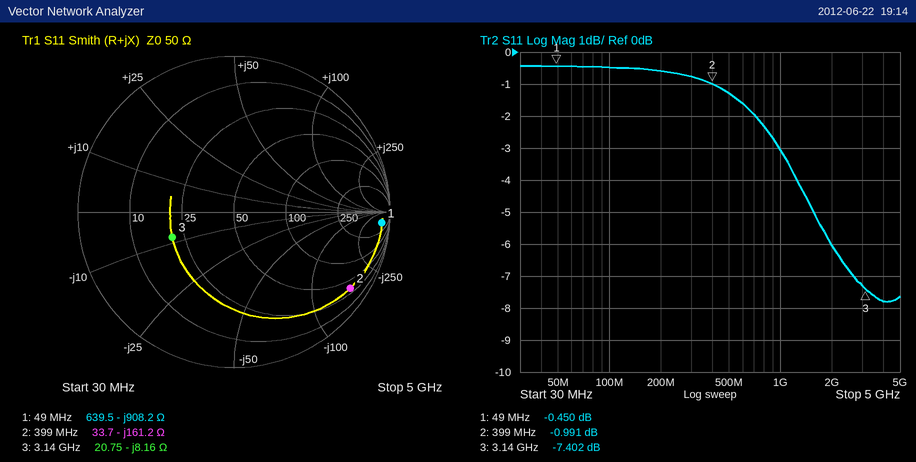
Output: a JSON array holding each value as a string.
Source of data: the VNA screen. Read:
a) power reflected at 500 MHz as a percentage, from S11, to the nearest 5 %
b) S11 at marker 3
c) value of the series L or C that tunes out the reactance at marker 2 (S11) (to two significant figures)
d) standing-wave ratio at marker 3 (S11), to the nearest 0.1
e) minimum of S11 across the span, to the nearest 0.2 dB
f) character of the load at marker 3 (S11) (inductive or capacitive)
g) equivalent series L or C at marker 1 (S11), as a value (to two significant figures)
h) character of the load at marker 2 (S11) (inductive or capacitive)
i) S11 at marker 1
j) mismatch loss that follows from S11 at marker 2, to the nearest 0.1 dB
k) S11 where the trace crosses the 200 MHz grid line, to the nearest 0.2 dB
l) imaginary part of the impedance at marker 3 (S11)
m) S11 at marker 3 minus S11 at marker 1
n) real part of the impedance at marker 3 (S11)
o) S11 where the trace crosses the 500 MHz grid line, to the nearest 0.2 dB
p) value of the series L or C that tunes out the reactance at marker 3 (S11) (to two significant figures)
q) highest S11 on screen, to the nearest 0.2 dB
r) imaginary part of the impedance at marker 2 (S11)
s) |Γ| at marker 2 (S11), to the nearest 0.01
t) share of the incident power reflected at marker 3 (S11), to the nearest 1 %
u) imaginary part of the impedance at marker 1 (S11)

["75 %", "-7.402 dB", "64 nH", "2.5", "-7.8 dB", "capacitive", "3.6 pF", "capacitive", "-0.450 dB", "6.9 dB", "-0.6 dB", "-8.16 Ω", "-6.952 dB", "20.75 Ω", "-1.2 dB", "410 pH", "-0.4 dB", "-161.2 Ω", "0.89", "18 %", "-908.2 Ω"]
